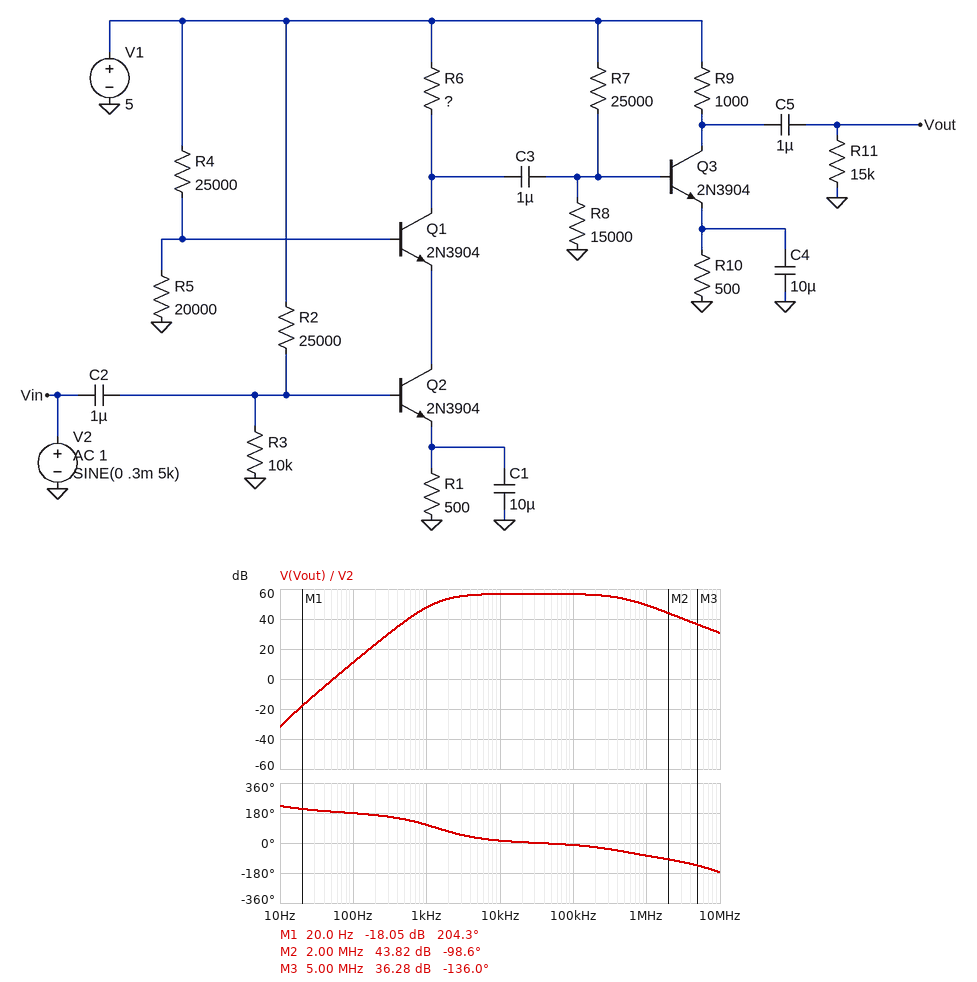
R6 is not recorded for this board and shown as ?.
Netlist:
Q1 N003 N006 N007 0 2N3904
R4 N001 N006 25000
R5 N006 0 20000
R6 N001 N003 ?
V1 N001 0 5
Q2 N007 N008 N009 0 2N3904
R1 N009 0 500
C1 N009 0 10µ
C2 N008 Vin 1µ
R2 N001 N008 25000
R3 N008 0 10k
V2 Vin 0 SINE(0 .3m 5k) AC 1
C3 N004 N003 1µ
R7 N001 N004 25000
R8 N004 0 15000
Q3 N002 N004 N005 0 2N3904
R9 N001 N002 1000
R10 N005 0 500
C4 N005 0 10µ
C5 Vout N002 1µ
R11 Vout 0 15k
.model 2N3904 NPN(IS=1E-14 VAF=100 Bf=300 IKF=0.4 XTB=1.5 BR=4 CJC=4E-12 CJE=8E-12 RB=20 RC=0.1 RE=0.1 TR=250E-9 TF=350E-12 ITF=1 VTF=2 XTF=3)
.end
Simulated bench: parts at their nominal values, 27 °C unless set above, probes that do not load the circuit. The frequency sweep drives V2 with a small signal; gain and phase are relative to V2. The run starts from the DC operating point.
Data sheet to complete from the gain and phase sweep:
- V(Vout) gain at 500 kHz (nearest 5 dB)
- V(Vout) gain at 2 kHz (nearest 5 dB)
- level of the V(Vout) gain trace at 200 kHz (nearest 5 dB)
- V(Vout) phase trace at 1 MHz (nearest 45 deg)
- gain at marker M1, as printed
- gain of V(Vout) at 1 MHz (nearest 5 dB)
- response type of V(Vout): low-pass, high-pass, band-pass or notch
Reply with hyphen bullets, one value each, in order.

- 55 dB
- 55 dB
- 55 dB
- -90 deg
- -18.05 dB
- 50 dB
- band-pass
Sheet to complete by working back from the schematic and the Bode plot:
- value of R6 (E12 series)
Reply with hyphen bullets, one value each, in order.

- 3.9 kΩ
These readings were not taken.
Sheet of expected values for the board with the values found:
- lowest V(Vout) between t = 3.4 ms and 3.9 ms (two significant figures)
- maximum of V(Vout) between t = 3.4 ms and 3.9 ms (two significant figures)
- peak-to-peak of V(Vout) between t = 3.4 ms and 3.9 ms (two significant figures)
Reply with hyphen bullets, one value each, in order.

- -200 mV
- 190 mV
- 390 mV
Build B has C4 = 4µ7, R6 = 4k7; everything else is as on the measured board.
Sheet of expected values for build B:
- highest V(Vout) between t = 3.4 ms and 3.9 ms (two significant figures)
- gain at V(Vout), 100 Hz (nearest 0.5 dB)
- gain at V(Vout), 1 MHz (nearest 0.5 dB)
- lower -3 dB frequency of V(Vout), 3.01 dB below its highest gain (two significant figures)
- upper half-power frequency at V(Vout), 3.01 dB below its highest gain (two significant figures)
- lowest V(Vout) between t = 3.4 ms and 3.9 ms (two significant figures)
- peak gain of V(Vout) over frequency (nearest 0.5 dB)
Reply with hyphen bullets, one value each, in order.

- 100 mV
- 1.5 dB
- 45.0 dB
- 3.3 kHz
- 470 kHz
- -110 mV
- 52.0 dB
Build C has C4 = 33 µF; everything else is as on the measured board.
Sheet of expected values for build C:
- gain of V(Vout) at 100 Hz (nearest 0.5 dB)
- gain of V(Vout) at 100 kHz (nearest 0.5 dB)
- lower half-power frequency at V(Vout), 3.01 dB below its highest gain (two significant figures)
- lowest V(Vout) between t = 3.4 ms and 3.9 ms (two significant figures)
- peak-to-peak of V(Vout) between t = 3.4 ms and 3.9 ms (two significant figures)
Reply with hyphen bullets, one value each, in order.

- 20.5 dB
- 56.5 dB
- 1.5 kHz
- -210 mV
- 400 mV
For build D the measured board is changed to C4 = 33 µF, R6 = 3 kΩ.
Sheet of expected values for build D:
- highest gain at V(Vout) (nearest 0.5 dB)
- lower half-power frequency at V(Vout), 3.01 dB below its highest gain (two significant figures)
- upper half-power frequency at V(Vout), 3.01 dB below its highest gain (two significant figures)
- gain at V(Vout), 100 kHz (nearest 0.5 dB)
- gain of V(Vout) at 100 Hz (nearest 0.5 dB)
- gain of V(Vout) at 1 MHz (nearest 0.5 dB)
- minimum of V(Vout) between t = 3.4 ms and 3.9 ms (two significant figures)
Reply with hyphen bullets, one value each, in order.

- 71.0 dB
- 1.2 kHz
- 440 kHz
- 70.5 dB
- 38.0 dB
- 63.0 dB
- -1.1 V
